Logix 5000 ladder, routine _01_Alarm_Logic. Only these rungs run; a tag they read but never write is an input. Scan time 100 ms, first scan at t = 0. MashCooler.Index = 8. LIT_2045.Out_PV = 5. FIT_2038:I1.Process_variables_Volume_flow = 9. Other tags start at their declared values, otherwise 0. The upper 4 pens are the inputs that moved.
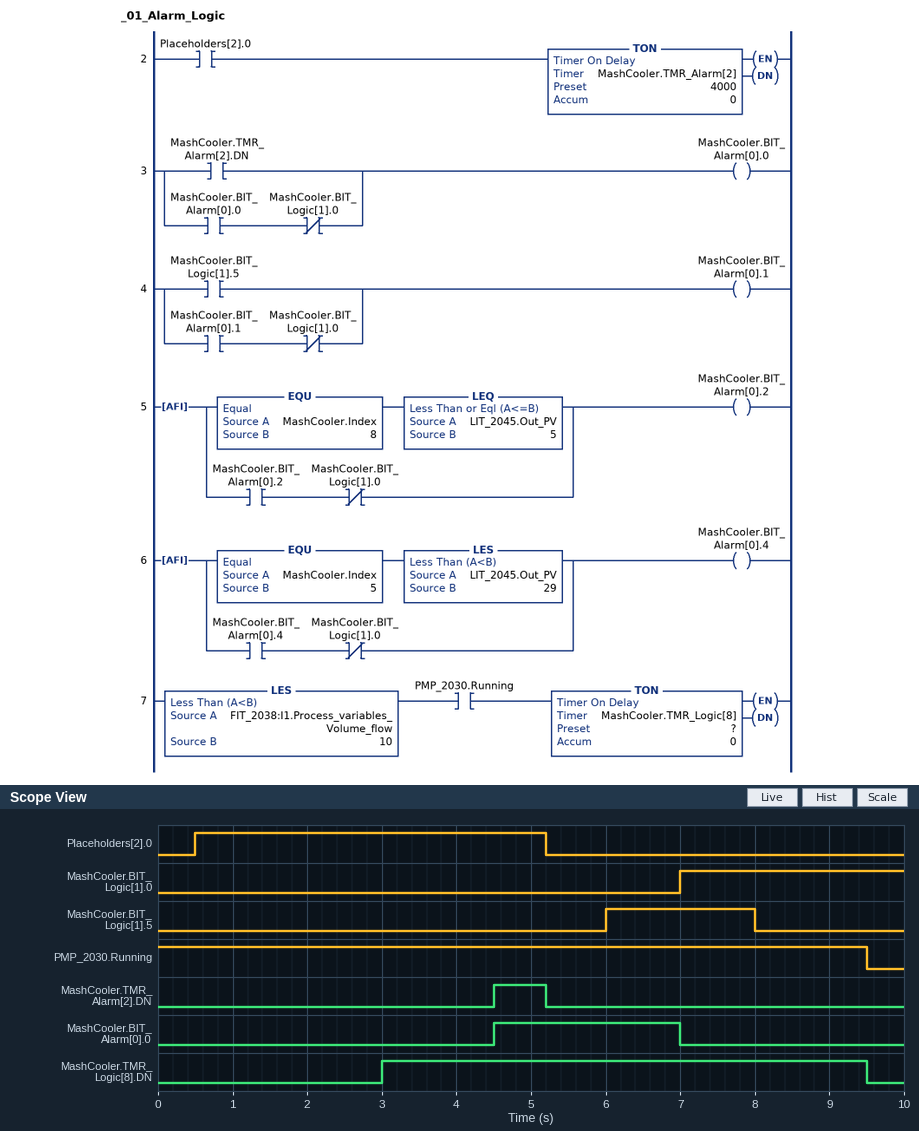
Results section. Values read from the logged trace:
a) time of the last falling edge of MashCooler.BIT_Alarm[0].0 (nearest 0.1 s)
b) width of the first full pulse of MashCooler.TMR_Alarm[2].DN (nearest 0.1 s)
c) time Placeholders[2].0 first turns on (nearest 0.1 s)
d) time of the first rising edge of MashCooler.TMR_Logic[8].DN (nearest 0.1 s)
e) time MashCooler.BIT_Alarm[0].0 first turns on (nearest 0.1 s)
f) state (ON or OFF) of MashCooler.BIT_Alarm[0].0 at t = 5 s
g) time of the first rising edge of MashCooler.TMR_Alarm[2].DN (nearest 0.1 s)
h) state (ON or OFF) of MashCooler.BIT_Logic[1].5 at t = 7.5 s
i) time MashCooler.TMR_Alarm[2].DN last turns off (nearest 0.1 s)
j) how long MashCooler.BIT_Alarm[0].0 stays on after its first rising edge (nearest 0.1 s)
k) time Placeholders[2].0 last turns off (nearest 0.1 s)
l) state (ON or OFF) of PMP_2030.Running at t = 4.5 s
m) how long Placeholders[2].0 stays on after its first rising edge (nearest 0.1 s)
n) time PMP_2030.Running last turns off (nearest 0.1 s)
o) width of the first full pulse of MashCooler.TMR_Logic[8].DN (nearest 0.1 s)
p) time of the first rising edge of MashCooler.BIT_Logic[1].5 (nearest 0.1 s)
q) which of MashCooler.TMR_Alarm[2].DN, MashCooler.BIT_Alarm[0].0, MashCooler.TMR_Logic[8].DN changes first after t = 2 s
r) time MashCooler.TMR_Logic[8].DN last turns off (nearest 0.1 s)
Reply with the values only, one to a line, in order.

7.0 s
0.7 s
0.5 s
3.0 s
4.5 s
ON
4.5 s
ON
5.2 s
2.5 s
5.2 s
ON
4.7 s
9.5 s
6.5 s
6.0 s
MashCooler.TMR_Logic[8].DN
9.5 s
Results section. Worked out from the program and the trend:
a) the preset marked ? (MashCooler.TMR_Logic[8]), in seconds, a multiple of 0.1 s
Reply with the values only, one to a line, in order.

3.0 s
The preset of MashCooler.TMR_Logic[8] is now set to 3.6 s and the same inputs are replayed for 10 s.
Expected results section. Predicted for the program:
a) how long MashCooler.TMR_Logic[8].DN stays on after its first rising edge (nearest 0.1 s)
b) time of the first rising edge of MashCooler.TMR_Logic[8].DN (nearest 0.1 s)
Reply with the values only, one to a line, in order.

5.9 s
3.6 s
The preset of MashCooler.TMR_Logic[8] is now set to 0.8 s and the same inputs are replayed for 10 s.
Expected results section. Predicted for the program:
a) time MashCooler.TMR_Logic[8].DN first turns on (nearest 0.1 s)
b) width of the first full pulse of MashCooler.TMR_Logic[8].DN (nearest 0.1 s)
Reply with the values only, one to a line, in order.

0.8 s
8.7 s
